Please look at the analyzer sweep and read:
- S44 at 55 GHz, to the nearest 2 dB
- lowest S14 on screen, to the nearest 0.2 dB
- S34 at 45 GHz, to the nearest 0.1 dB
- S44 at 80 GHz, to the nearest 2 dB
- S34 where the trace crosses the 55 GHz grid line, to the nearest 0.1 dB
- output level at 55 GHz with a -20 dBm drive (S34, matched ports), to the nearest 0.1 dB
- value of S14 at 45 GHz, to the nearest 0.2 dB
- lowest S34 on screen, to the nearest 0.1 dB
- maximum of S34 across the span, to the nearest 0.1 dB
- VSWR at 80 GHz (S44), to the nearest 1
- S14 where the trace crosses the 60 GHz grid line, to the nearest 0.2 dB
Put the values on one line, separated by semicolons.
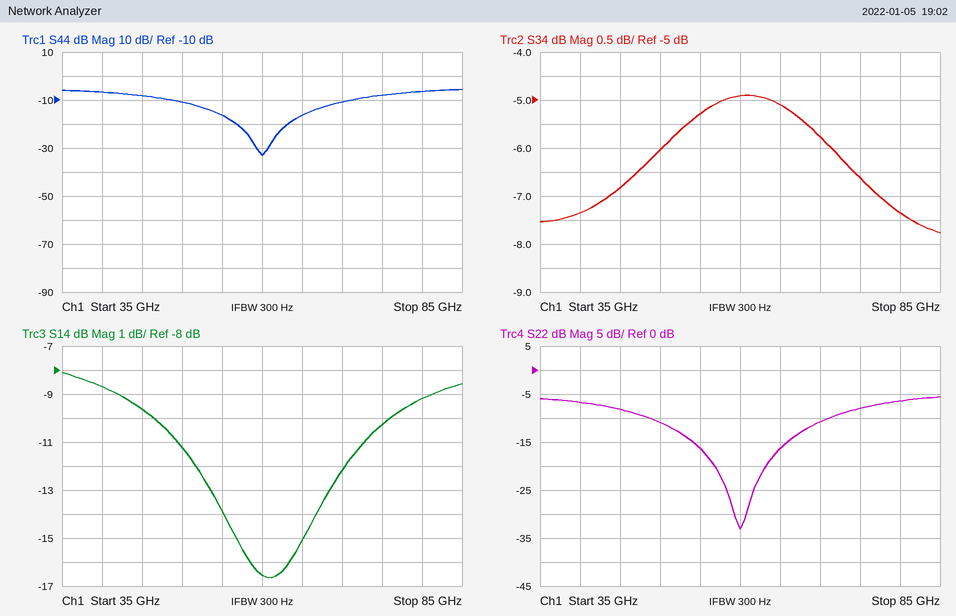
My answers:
-16 dB; -16.6 dB; -6.8 dB; -6 dB; -5.3 dB; -25.3 dBm; -9.6 dB; -7.8 dB; -4.9 dB; 3; -16.6 dB
